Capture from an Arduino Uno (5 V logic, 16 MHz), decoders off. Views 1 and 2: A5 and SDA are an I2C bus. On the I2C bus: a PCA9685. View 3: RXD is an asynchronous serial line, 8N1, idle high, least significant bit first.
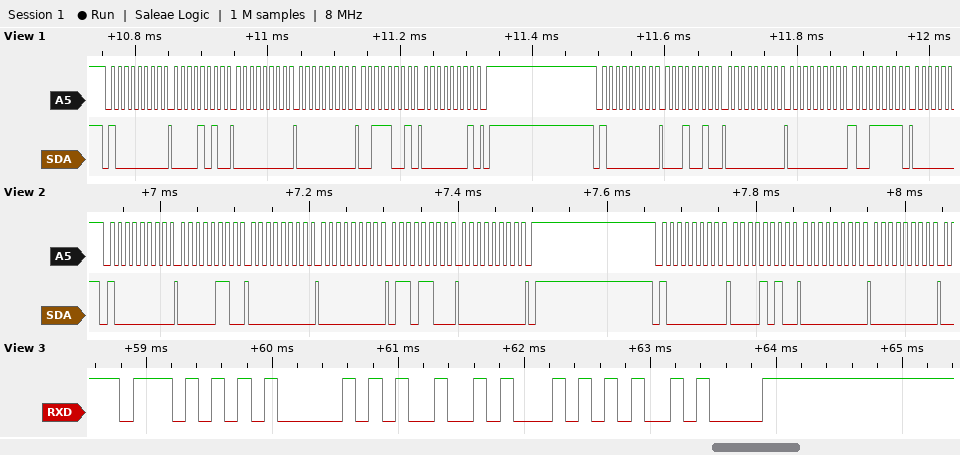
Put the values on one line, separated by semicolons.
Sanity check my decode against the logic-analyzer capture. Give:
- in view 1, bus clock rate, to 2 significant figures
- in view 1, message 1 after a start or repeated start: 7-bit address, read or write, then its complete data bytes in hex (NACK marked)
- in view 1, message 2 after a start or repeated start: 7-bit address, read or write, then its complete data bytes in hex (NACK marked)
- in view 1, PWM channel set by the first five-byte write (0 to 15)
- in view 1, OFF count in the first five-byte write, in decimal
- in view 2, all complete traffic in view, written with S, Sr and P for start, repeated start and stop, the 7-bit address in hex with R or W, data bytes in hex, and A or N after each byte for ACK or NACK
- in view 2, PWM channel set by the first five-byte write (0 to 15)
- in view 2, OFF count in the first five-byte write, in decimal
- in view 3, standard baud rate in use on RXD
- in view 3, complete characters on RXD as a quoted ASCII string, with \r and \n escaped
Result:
100 kHz; 0x40 write: 0A 00 00 39 01; 0x40 write: 12 00 00 9F; 1; 313; S 40W A 06 A 00 A 00 A 6C A 00 A P S 40W A 0A A 00 A 00 A; 0; 108; 9600 baud; "WAIT\n"
